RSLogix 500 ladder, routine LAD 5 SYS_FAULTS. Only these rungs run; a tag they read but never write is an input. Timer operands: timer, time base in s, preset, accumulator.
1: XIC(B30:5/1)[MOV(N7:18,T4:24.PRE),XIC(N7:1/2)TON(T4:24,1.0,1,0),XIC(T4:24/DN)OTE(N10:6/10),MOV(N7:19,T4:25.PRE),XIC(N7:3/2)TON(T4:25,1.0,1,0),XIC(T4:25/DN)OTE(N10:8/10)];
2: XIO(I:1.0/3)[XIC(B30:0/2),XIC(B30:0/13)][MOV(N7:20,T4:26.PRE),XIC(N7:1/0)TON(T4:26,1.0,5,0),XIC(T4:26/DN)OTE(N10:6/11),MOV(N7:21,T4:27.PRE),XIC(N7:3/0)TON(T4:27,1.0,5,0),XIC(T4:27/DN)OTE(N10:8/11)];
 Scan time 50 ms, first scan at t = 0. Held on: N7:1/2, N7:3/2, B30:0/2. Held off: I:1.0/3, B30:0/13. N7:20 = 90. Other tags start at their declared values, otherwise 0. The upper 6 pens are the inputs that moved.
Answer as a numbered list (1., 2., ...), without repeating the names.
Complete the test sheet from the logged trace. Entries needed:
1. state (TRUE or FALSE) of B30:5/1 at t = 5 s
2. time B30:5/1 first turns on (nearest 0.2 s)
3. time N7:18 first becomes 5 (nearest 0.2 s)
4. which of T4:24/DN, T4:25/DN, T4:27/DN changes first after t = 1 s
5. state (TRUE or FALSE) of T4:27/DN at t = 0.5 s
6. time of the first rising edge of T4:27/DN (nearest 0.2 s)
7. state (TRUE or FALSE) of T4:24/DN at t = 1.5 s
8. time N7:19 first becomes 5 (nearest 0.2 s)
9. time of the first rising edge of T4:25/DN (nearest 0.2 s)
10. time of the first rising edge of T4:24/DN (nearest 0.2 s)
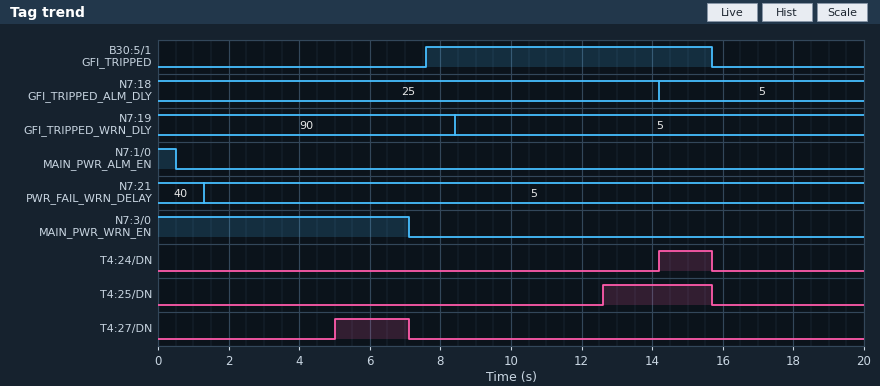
1. FALSE
2. 7.6 s
3. 14.2 s
4. T4:27/DN
5. FALSE
6. 5.0 s
7. FALSE
8. 8.4 s
9. 12.6 s
10. 14.2 s
